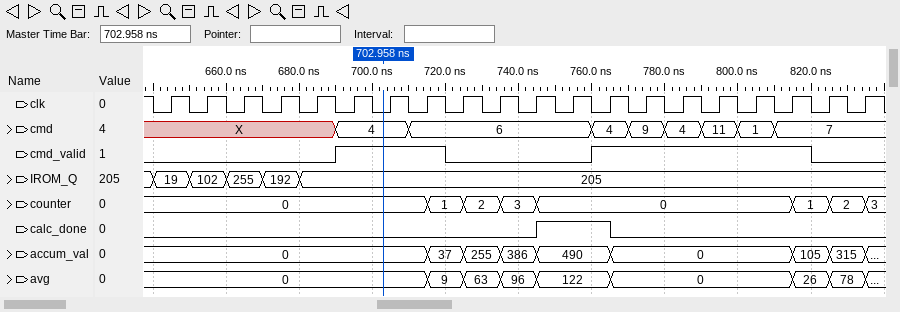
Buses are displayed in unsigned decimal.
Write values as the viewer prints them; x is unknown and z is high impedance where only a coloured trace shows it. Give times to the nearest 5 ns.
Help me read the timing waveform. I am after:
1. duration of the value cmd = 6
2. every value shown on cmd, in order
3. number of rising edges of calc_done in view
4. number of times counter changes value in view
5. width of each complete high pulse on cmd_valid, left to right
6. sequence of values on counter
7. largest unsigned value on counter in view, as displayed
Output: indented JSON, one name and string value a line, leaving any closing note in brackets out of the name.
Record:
{
  "duration of the value cmd = 6": "50 ns",
  "every value shown on cmd, in order": "X, 4, 6, 4, 9, 4, 11, 1, 7",
  "number of rising edges of calc_done in view": "1",
  "number of times counter changes value in view": "7",
  "width of each complete high pulse on cmd_valid, left to right": "30 ns, 60 ns",
  "sequence of values on counter": "0, 1, 2, 3, 0, 1, 2, 3",
  "largest unsigned value on counter in view, as displayed": "3"
}
